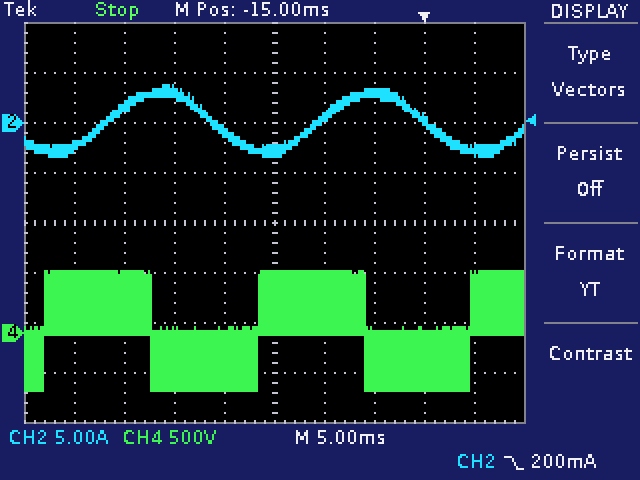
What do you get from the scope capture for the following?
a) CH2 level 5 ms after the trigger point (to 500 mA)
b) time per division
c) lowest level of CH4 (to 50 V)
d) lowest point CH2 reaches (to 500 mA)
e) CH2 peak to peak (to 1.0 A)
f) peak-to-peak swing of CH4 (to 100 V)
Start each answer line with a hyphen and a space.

- -3.0 A
- 5 ms
- -600 V
- -3.5 A
- 7.0 A
- 1.20 kV
